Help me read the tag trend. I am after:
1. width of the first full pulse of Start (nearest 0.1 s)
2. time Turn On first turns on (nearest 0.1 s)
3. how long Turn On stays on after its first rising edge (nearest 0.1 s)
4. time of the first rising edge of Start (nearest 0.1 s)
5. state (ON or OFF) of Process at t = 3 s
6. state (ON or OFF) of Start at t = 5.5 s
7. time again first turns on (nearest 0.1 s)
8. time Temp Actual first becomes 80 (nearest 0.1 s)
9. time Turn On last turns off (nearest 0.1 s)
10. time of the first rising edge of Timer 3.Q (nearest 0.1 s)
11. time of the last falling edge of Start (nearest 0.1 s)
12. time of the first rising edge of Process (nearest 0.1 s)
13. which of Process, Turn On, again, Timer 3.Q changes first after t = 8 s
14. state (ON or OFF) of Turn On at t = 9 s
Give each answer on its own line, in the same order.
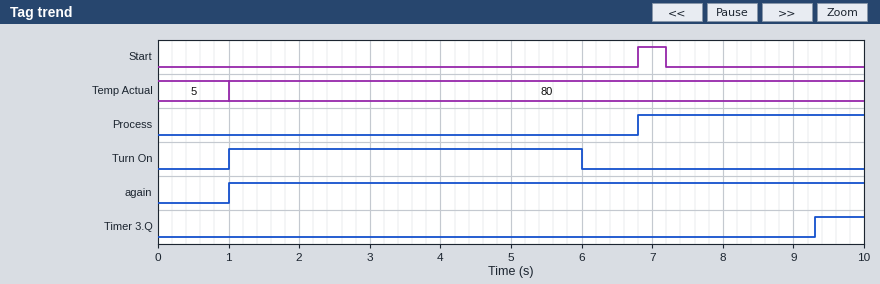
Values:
0.4 s
1.0 s
5.0 s
6.8 s
OFF
OFF
1.0 s
1.0 s
6.0 s
9.3 s
7.2 s
6.8 s
Timer 3.Q
OFF
